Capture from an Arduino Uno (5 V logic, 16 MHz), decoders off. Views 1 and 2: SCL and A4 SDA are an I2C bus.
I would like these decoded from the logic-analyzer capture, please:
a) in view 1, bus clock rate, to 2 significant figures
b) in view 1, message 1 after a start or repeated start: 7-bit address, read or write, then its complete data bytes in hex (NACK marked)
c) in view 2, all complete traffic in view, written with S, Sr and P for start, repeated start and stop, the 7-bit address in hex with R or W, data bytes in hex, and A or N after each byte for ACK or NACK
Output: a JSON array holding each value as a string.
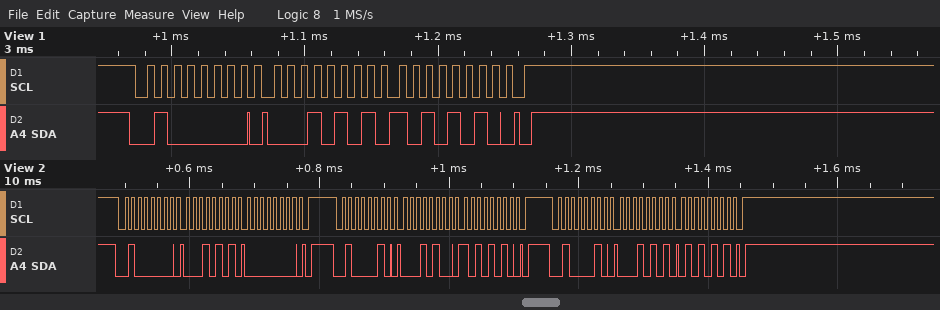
["100 kHz", "0x20 write: 15 AA", "S 20W A 15 A 00 A P S 21W A 14 A AA A P S 21W A 15 A 55 A P"]
